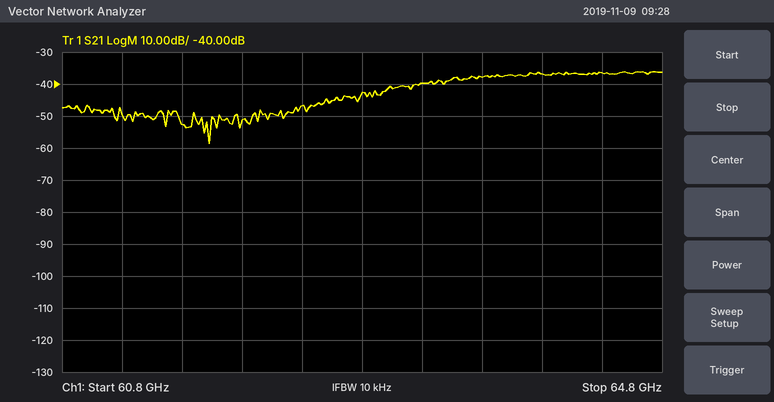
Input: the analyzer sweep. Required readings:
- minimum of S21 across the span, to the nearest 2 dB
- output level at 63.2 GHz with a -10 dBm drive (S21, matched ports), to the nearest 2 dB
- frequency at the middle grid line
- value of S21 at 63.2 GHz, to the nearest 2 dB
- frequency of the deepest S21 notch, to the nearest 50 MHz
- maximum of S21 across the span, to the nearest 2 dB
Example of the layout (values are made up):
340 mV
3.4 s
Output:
-58 dB
-50 dBm
62.8 GHz
-40 dB
61.80 GHz
-36 dB
